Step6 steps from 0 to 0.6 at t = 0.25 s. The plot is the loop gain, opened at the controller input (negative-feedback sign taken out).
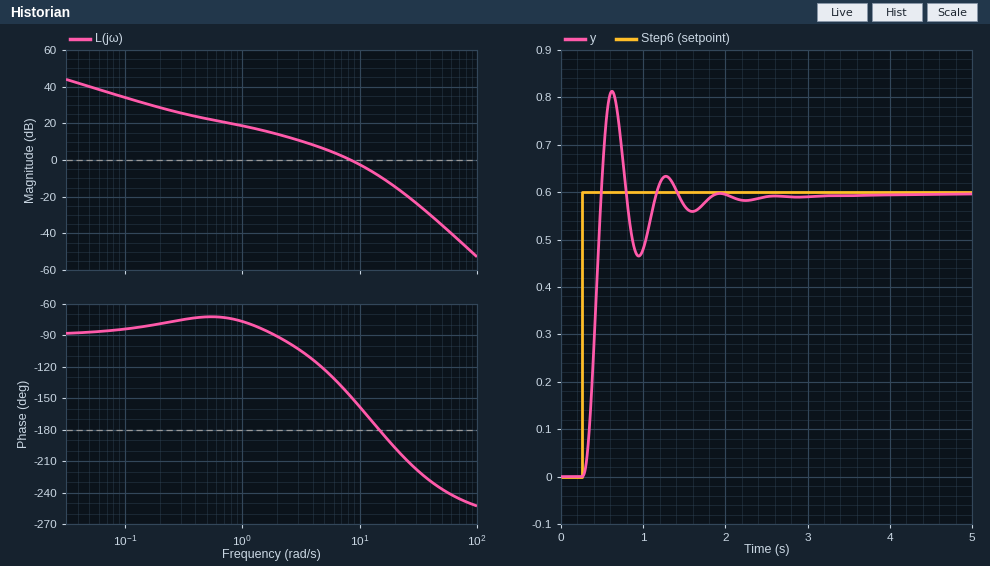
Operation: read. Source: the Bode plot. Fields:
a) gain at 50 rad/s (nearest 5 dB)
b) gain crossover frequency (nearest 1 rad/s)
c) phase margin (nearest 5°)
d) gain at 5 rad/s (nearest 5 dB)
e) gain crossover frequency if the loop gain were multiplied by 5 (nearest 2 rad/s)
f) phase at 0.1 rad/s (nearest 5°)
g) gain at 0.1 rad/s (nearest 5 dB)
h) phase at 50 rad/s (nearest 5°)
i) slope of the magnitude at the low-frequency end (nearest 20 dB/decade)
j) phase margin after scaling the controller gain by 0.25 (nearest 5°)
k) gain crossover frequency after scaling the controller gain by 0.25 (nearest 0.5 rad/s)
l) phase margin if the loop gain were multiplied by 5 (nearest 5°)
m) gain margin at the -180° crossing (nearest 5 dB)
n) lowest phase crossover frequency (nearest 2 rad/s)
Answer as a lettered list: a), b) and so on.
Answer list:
a) -35 dB
b) 8 rad/s
c) 30°
d) 5 dB
e) 20 rad/s
f) -85°
g) 35 dB
h) -235°
i) -20 dB/decade
j) 80°
k) 2.5 rad/s
l) -15°
m) 10 dB
n) 14 rad/s
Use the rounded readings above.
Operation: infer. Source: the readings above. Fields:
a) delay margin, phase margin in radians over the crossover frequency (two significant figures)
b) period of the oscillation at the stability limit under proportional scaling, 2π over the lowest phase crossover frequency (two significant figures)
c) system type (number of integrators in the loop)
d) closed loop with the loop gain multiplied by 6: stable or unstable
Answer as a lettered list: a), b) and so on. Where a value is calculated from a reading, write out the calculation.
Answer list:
a) 30 × π / 180 / 8 = 0.065 s
b) 2π / 14 = 0.45 s
c) 1
d) unstable
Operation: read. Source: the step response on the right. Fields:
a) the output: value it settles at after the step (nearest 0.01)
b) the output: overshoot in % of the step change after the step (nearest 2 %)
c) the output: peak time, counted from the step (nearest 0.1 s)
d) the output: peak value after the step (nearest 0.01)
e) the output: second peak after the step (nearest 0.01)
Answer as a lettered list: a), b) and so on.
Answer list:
a) 0.60
b) 36 %
c) 0.4 s
d) 0.81
e) 0.63
